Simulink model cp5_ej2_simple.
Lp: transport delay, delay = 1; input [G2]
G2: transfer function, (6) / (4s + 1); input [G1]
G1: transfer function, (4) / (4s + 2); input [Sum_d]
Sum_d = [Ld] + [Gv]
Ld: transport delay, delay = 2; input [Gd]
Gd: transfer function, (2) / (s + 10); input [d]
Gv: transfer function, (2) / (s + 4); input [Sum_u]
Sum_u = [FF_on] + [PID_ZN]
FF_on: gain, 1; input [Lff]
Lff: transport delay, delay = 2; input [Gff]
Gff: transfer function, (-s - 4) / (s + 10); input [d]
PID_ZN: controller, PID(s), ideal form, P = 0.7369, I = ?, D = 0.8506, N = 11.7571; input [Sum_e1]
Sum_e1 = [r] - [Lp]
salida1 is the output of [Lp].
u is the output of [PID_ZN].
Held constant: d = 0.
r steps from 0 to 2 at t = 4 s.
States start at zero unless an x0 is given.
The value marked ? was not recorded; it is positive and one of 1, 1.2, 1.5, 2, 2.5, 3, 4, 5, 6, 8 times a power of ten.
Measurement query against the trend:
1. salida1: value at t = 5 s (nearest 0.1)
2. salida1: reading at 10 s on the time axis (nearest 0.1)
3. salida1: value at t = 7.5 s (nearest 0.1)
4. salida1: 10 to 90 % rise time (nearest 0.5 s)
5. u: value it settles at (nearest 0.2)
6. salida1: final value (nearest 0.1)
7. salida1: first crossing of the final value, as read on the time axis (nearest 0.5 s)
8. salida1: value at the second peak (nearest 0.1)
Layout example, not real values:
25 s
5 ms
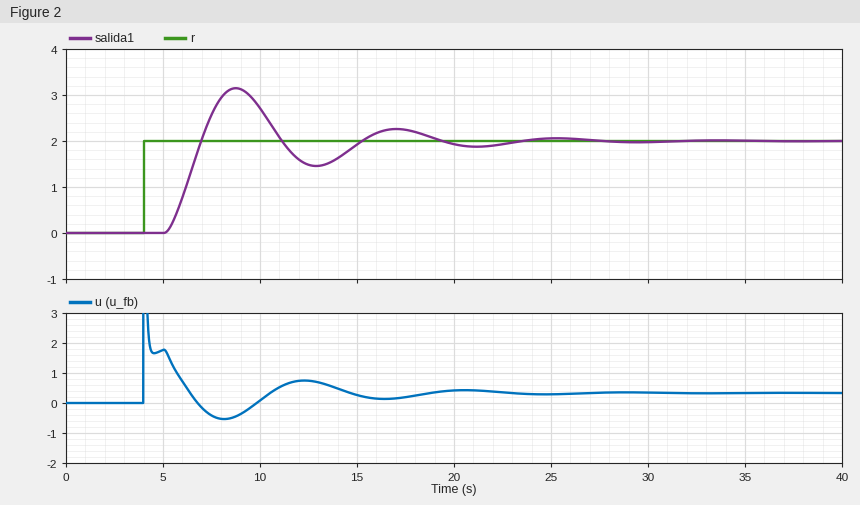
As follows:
0.0
2.7
2.6
1.5 s
0.4
2.0
7.0 s
2.3
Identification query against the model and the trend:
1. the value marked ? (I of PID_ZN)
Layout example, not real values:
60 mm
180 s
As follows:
0.2
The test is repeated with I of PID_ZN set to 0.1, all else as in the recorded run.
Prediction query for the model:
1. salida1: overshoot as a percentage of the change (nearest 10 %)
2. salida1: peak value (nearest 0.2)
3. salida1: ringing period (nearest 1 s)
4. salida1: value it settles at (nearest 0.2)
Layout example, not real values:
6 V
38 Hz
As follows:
40 %
2.8
8 s
2.0
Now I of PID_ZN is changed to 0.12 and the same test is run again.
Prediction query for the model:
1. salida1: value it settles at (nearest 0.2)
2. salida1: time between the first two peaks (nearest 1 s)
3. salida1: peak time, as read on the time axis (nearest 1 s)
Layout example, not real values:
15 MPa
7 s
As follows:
2.0
8 s
9 s
